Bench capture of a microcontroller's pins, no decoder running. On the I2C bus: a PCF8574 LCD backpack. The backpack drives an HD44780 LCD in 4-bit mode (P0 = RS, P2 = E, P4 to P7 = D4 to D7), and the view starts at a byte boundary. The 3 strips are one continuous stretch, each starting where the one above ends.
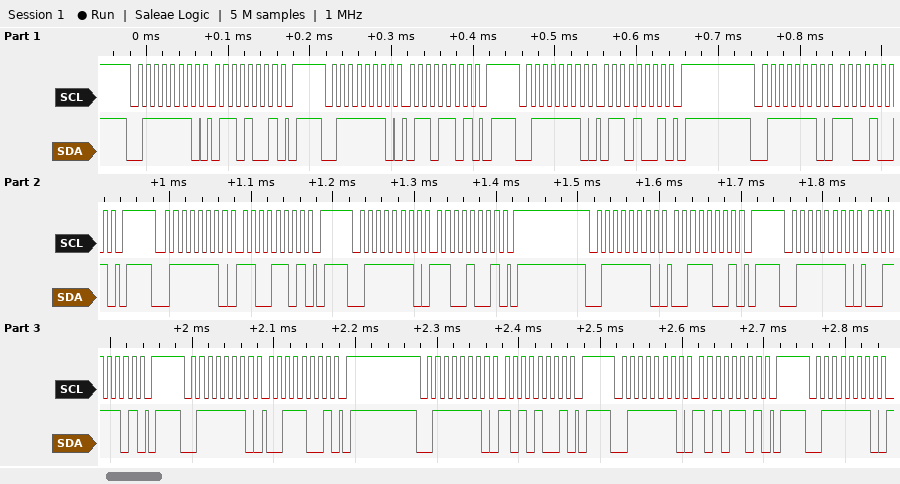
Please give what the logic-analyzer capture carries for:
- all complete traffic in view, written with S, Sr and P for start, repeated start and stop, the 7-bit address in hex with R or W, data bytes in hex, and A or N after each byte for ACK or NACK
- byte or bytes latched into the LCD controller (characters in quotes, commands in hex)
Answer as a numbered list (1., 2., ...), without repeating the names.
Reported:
1. S 3FW A 69 A P S 3FW A 6D A P S 3FW A 69 A P S 3FW A C9 A P S 3FW A CD A P S 3FW A C9 A P S 3FW A 39 A P S 3FW A 3D A P S 3FW A 39 A P S 3FW A A9 A P S 3FW A AD A P S 3FW A
2. 'l'
